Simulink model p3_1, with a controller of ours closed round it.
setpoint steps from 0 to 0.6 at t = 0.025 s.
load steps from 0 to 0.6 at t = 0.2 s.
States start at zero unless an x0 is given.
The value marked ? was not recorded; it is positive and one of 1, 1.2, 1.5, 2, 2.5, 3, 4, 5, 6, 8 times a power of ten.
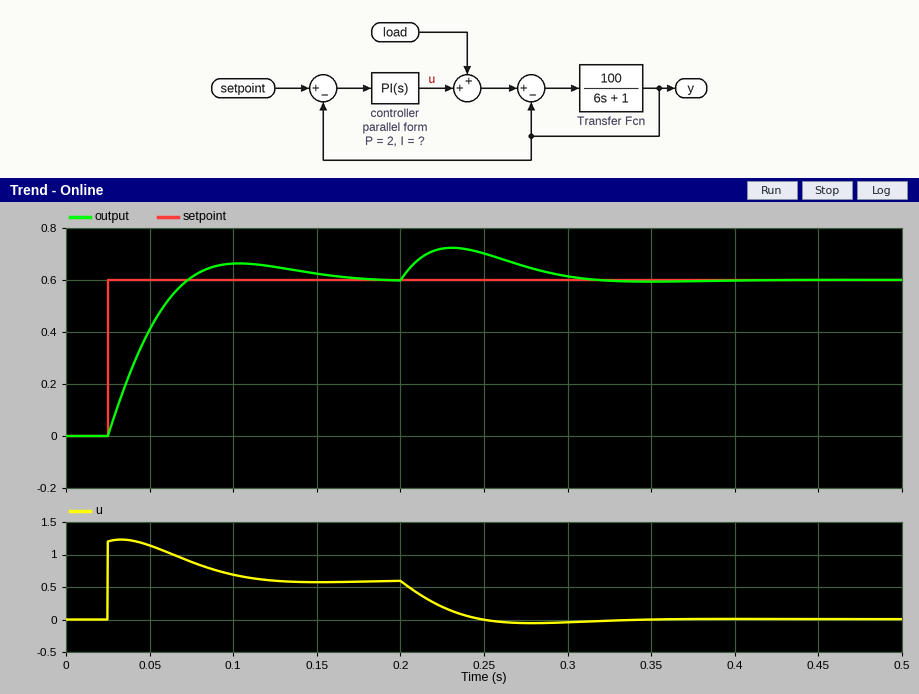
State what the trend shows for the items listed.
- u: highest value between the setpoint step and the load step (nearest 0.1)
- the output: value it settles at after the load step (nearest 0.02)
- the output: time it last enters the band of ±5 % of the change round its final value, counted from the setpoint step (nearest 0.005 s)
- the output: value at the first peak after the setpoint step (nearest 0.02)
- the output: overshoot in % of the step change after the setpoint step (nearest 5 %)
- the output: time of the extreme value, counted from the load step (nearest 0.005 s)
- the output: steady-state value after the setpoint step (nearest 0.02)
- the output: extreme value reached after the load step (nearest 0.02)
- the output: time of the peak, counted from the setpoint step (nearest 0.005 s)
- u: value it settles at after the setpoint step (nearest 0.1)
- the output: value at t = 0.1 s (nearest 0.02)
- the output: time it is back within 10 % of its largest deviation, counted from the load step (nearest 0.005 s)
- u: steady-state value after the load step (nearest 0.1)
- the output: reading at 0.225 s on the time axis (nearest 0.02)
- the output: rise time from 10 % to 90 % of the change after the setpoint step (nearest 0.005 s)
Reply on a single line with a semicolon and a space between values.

1.2; 0.60; 0.120 s; 0.66; 10 %; 0.030 s; 0.60; 0.72; 0.080 s; 0.6; 0.66; 0.100 s; 0.0; 0.72; 0.035 s
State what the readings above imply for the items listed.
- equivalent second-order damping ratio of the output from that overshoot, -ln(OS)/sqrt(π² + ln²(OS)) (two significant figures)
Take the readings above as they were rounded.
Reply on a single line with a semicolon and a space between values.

0.59
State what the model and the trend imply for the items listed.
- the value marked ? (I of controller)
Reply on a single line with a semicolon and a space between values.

80
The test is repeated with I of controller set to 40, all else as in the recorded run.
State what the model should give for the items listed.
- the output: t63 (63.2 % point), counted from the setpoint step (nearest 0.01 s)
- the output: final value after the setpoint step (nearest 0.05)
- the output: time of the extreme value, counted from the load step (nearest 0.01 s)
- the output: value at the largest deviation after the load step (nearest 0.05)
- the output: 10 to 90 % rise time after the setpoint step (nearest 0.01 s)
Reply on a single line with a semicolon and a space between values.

0.03 s; 0.60; 0.04 s; 0.75; 0.06 s
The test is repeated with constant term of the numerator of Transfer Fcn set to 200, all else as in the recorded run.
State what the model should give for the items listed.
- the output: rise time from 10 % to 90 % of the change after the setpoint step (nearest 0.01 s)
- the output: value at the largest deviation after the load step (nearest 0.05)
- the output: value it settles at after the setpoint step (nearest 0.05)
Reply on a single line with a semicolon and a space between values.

0.03 s; 0.75; 0.60
